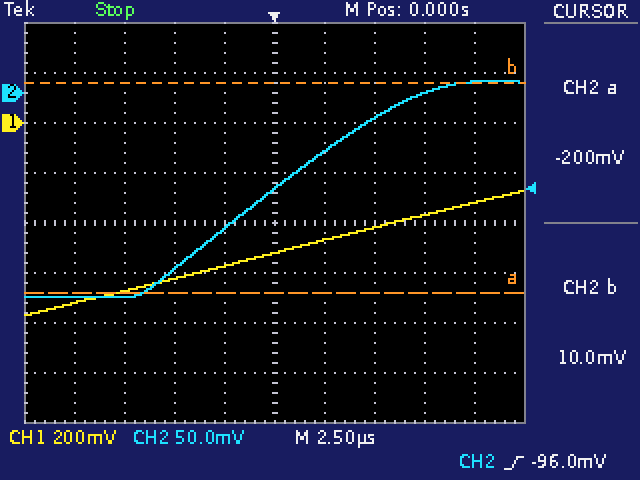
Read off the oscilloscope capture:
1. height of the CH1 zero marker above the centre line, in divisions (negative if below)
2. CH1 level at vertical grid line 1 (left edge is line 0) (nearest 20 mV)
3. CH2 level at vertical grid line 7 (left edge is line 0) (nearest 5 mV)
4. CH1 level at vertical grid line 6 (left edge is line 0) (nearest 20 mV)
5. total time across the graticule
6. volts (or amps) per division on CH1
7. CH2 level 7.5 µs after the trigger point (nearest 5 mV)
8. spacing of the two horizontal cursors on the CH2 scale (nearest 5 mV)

+2.0 div
-720 mV
-25 mV
-460 mV
25 µs
200 mV
0 mV
210 mV
